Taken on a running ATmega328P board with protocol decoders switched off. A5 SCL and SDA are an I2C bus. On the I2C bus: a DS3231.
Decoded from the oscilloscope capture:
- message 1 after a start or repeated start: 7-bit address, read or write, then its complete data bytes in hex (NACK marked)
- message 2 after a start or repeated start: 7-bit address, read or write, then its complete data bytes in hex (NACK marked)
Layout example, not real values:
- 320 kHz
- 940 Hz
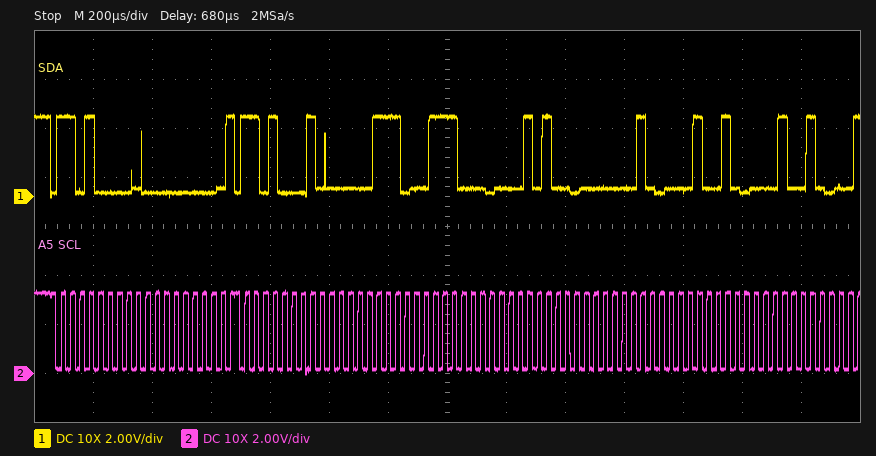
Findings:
- 0x68 write: 00
- 0x68 read: 07 38 14 02 12 12
